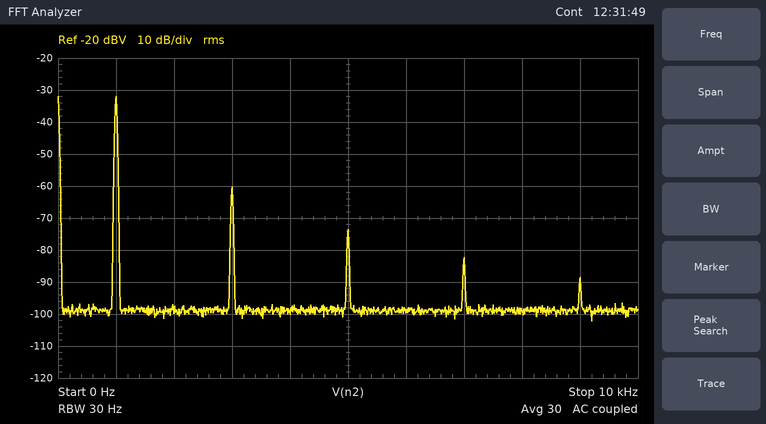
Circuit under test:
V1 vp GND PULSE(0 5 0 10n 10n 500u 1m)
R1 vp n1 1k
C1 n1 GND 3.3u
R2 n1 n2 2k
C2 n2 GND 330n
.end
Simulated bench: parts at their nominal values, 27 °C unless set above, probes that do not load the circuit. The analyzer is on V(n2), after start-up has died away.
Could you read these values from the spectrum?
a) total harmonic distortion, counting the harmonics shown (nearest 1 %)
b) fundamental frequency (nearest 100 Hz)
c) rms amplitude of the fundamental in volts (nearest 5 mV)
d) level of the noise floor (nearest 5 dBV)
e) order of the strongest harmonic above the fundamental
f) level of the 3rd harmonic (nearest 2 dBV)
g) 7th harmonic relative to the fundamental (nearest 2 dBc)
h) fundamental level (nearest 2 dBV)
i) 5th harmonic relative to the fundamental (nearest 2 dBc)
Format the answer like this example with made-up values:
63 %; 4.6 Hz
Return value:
4 %; 1.0 kHz; 25 mV; -100 dBV; 3; -60 dBV; -50 dBc; -32 dBV; -42 dBc
